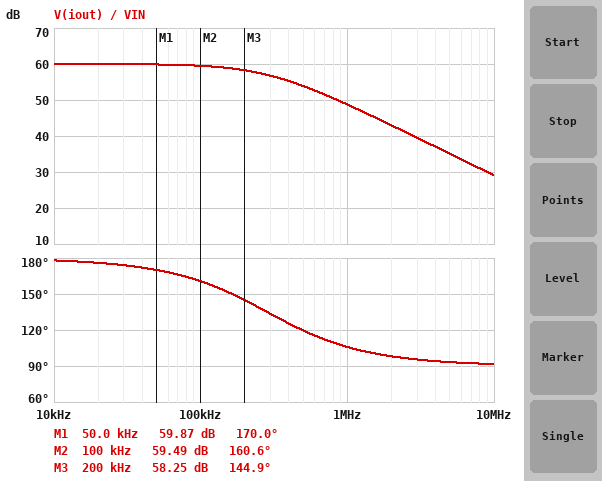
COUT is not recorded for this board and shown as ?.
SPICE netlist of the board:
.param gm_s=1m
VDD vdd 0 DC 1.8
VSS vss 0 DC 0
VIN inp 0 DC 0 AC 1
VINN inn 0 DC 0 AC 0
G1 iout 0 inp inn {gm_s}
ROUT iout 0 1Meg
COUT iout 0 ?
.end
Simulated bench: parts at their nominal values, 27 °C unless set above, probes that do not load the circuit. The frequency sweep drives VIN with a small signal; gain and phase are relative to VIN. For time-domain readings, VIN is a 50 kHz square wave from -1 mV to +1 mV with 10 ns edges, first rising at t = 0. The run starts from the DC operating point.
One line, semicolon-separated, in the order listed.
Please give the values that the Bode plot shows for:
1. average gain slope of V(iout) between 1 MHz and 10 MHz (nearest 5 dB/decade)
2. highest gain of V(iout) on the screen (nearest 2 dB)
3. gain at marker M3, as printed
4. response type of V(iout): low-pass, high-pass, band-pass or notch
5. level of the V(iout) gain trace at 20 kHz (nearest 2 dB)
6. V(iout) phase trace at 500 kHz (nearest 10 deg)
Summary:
-20 dB/decade; 60 dB; 58.25 dB; low-pass; 60 dB; 120 deg
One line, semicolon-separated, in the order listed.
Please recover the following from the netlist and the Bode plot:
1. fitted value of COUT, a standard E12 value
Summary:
560 fF
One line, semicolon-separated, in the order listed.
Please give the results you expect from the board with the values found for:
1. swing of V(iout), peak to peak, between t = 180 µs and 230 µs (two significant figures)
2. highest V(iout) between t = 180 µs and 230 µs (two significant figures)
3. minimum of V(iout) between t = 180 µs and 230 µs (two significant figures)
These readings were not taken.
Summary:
2.0 V; 1.0 V; -1.0 V
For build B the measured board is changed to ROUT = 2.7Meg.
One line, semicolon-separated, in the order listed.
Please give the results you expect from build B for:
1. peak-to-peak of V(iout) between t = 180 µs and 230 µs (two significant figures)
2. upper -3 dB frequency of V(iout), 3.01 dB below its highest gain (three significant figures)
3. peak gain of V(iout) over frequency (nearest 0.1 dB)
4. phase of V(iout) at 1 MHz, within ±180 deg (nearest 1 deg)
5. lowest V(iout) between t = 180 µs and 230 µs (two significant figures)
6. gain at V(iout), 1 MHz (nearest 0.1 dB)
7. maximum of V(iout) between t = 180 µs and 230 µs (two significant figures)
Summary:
5.4 V; 105 kHz; 68.6 dB; 96 deg; -2.7 V; 49.0 dB; 2.7 V
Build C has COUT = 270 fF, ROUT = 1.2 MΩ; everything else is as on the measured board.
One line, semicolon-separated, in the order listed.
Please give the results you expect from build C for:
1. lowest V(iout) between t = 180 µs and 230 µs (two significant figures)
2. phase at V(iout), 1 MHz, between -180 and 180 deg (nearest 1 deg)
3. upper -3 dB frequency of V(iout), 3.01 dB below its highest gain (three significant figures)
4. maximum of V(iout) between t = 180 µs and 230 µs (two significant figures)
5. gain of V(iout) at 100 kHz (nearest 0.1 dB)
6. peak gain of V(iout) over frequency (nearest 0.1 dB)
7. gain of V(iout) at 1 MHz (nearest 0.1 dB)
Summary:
-1.2 V; 116 deg; 491 kHz; 1.2 V; 61.4 dB; 61.6 dB; 54.5 dB
